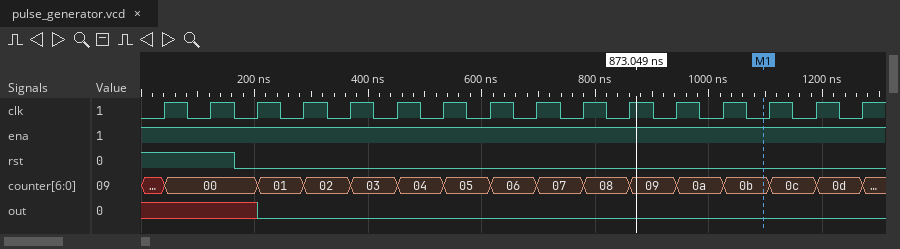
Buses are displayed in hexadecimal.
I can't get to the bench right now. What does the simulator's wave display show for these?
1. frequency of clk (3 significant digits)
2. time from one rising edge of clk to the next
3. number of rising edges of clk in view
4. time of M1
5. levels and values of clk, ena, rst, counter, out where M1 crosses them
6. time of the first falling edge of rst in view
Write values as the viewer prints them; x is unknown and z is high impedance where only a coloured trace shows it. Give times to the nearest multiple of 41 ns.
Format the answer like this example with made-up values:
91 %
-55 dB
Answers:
12.2 MHz
82 ns
16
1107 ns
clk=0, ena=1, rst=0, counter=0b, out=0
164 ns
